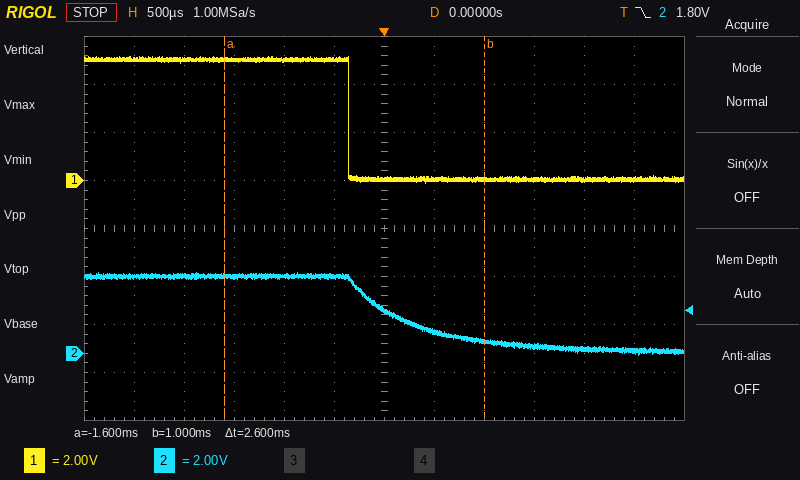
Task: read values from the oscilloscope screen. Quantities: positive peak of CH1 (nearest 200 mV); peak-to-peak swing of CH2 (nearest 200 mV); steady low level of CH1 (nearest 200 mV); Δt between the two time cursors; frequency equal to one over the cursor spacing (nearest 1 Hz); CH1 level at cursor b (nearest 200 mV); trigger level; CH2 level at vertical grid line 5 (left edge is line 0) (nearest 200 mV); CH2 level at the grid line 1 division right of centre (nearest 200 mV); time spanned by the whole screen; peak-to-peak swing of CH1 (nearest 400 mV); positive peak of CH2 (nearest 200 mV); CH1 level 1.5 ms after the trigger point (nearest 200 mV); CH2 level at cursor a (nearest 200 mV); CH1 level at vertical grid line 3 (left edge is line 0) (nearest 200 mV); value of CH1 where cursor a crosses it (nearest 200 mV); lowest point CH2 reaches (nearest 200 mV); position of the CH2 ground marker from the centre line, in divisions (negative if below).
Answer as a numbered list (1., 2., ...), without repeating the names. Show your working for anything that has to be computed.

1. 5.2 V
2. 3.4 V − (0.0 V) = 3.4 V
3. 0.0 V
4. 2.6 ms
5. 1 / 2.6 ms ≈ 385 Hz
6. 0.0 V
7. 1.80 V
8. 3.2 V
9. 1.0 V
10. 6 ms
11. 5.2 V
12. 3.4 V
13. 0.0 V
14. 3.2 V
15. 5.0 V
16. 5.0 V
17. 0.0 V
18. -2.6 div
